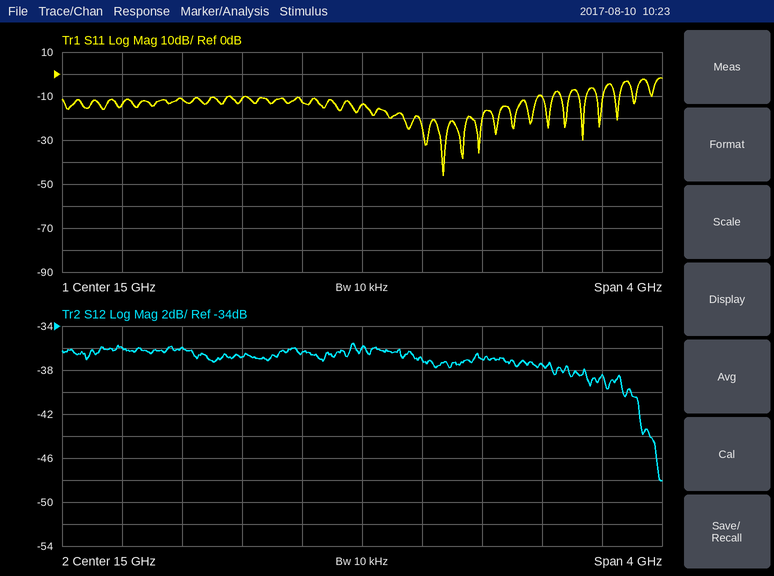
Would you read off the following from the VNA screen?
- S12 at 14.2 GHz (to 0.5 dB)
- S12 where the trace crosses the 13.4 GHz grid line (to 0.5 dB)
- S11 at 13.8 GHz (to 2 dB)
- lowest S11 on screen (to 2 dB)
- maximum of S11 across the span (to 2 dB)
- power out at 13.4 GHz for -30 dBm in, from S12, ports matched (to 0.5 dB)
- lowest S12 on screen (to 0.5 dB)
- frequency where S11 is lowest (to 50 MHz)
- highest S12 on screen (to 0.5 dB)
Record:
-37.0 dB
-36.0 dB
-12 dB
-46 dB
-2 dB
-66.0 dBm
-48.0 dB
15.55 GHz
-35.5 dB
